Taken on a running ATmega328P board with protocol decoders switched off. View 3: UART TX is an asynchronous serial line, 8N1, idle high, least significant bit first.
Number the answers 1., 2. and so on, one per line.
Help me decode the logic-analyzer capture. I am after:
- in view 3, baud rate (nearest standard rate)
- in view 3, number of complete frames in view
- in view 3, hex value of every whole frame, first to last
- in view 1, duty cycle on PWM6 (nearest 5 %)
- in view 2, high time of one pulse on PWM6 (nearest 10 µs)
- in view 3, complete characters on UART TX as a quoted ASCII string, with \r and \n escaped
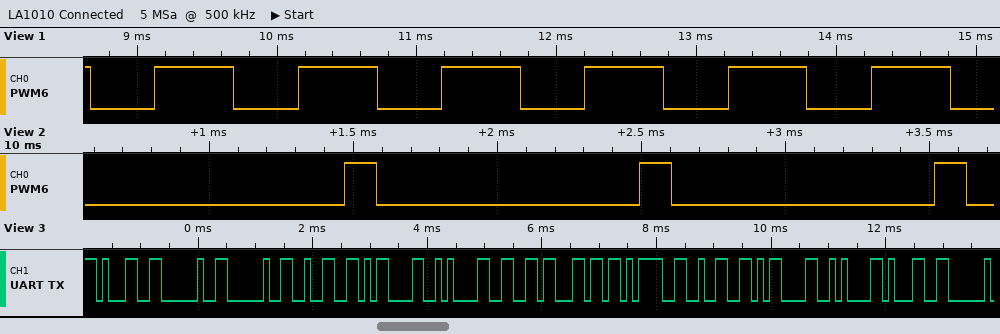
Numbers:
1. 9600 baud
2. 13
3. 31 20 20 32 0D 0A 66 6C 3D 32 0D 0A 31
4. 55 %
5. 110 µs
6. "1  2\r\nfl=2\r\n1"
